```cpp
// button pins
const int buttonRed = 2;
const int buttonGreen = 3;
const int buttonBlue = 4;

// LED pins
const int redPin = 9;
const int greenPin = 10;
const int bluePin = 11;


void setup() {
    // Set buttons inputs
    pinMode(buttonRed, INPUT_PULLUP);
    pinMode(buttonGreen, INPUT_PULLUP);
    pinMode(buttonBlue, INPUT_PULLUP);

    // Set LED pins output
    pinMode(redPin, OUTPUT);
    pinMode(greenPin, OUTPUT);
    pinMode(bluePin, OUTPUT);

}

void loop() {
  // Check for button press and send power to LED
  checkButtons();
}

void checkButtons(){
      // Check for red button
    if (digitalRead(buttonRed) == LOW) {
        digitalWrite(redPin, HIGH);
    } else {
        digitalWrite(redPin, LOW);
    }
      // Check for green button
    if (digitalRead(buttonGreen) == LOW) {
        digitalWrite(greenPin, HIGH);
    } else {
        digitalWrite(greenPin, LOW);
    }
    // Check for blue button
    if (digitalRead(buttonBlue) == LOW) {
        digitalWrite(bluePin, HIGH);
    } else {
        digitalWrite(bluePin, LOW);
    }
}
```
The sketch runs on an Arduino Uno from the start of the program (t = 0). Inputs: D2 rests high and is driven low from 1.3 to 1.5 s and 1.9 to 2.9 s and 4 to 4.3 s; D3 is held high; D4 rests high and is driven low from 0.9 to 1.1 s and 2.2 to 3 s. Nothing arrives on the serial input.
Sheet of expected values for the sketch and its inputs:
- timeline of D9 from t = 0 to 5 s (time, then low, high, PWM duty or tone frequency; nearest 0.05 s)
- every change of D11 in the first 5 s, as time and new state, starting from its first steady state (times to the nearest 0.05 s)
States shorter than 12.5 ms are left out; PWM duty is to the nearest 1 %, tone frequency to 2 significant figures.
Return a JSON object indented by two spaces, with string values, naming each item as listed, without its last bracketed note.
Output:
{
  "timeline of D9 from t = 0 to 5 s": "0 s low; 1.3 s high; 1.5 s low; 1.9 s high; 2.9 s low; 4 s high; 4.3 s low",
  "every change of D11 in the first 5 s, as time and new state, starting from its first steady state": "0 s low; 0.9 s high; 1.1 s low; 2.2 s high; 3 s low"
}
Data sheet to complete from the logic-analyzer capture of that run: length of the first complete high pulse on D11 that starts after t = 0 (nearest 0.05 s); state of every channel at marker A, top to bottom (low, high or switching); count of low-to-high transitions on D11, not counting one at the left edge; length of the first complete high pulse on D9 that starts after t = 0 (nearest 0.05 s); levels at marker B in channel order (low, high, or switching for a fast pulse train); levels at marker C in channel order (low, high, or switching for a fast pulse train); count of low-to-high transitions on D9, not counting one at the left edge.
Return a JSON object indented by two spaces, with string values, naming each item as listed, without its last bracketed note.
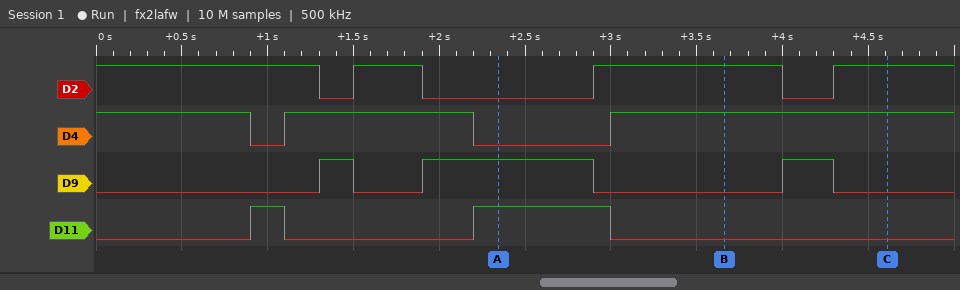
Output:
{
  "length of the first complete high pulse on D11 that starts after t = 0": "0.20 s",
  "state of every channel at marker A, top to bottom": "D2 low, D4 low, D9 high, D11 high",
  "count of low-to-high transitions on D11, not counting one at the left edge": "2",
  "length of the first complete high pulse on D9 that starts after t = 0": "0.20 s",
  "levels at marker B in channel order": "D2 high, D4 high, D9 low, D11 low",
  "levels at marker C in channel order": "D2 high, D4 high, D9 low, D11 low",
  "count of low-to-high transitions on D9, not counting one at the left edge": "3"
}
